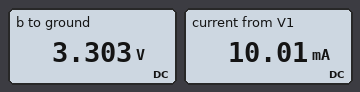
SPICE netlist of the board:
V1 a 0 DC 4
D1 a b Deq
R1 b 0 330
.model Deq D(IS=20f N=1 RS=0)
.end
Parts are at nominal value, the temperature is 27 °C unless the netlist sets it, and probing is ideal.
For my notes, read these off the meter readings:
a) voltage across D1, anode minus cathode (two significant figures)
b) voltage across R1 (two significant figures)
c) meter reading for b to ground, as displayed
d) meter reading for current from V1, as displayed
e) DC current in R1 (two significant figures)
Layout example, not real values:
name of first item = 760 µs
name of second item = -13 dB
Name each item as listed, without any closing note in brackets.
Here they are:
voltage across D1, anode minus cathode = 700 mV
voltage across R1 = 3.3 V
meter reading for b to ground, as displayed = 3.303 V
meter reading for current from V1, as displayed = 10.01 mA
DC current in R1 = 10 mA
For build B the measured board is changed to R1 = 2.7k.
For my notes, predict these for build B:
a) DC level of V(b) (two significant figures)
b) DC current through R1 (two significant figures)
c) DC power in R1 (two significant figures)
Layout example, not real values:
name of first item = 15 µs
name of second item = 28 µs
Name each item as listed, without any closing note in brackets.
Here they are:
DC level of V(b) = 3.4 V
DC current through R1 = 1.2 mA
DC power in R1 = 4.2 mW
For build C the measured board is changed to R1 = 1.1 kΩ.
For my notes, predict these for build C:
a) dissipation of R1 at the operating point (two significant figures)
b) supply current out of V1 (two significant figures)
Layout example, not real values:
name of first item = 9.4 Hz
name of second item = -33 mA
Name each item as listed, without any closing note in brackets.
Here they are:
dissipation of R1 at the operating point = 10 mW
supply current out of V1 = 3.0 mA
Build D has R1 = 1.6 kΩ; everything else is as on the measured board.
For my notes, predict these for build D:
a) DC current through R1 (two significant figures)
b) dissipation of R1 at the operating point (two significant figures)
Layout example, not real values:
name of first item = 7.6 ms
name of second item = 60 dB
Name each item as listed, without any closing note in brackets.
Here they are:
DC current through R1 = 2.1 mA
dissipation of R1 at the operating point = 7.0 mW
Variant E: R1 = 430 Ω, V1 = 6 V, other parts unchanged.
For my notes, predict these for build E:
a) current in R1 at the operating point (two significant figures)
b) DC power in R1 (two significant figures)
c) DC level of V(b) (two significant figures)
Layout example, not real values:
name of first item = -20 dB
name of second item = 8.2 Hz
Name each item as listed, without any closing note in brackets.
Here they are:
current in R1 at the operating point = 12 mA
DC power in R1 = 65 mW
DC level of V(b) = 5.3 V
